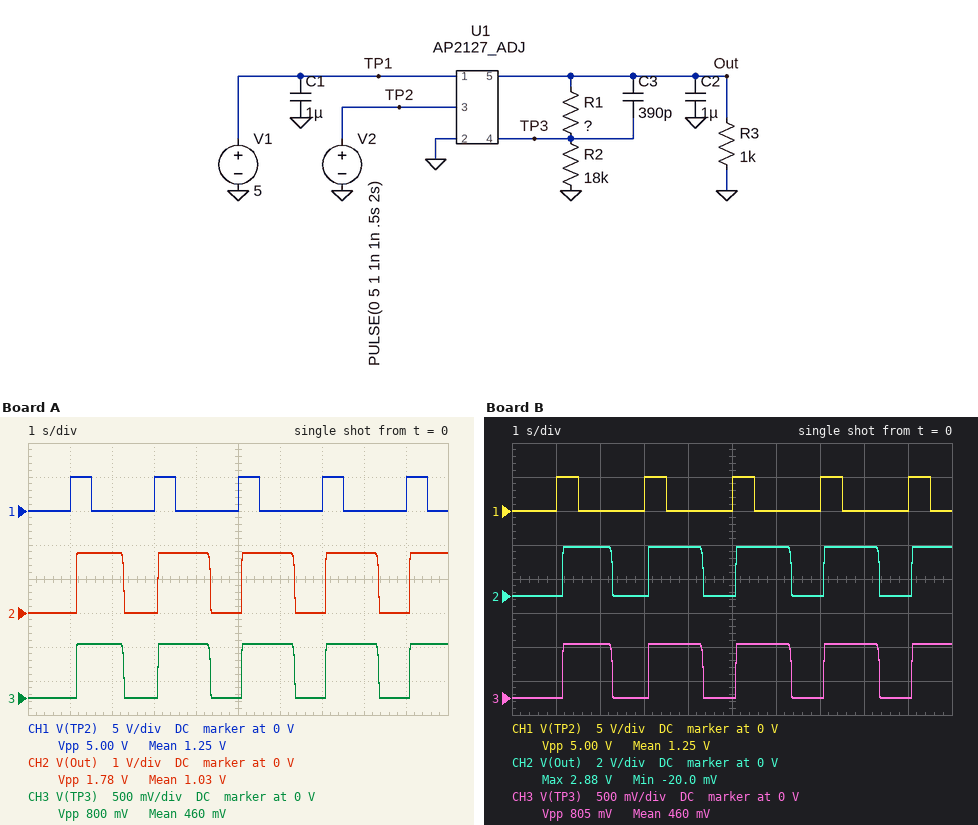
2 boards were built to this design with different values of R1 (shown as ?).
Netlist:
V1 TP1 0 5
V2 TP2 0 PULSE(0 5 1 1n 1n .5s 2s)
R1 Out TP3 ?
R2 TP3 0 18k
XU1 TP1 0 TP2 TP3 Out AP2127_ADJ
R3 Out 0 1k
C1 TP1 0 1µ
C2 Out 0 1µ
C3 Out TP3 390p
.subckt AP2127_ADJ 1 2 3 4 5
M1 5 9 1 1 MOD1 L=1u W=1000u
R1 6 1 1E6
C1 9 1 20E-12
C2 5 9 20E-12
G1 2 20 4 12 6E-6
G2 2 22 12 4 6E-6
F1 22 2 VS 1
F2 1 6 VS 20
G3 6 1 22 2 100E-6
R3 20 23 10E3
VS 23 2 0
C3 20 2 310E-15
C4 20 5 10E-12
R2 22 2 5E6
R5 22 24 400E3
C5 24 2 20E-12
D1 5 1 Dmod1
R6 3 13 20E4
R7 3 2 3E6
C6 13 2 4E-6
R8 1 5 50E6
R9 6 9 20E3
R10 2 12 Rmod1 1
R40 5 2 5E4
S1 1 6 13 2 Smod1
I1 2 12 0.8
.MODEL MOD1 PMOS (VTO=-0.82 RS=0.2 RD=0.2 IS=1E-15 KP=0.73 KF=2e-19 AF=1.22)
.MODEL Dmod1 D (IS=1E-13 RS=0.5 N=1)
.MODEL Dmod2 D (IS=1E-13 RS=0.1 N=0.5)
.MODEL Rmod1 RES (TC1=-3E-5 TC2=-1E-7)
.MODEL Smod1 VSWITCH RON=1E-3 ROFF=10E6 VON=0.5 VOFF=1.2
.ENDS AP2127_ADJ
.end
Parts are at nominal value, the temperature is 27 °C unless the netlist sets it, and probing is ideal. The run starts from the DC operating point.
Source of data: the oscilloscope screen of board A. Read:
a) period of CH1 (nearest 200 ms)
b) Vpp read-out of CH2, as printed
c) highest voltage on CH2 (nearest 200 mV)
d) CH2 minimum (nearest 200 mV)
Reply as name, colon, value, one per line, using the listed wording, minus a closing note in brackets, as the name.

period of CH1: 2.0 s
Vpp read-out of CH2, as printed: 1.78 V
highest voltage on CH2: 1.8 V
CH2 minimum: 0 V
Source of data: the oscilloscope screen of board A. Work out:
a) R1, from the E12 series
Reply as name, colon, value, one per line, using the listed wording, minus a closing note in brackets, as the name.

R1, from the E12 series: 22 kΩ
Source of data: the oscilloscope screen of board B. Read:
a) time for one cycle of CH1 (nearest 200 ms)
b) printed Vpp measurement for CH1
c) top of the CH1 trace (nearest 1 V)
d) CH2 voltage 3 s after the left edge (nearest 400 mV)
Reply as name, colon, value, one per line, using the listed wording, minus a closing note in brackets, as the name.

time for one cycle of CH1: 2.0 s
printed Vpp measurement for CH1: 5.00 V
top of the CH1 trace: 5 V
CH2 voltage 3 s after the left edge: 0 V
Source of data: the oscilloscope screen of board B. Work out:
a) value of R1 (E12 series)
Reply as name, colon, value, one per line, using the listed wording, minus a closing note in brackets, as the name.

value of R1: 47 kΩ
